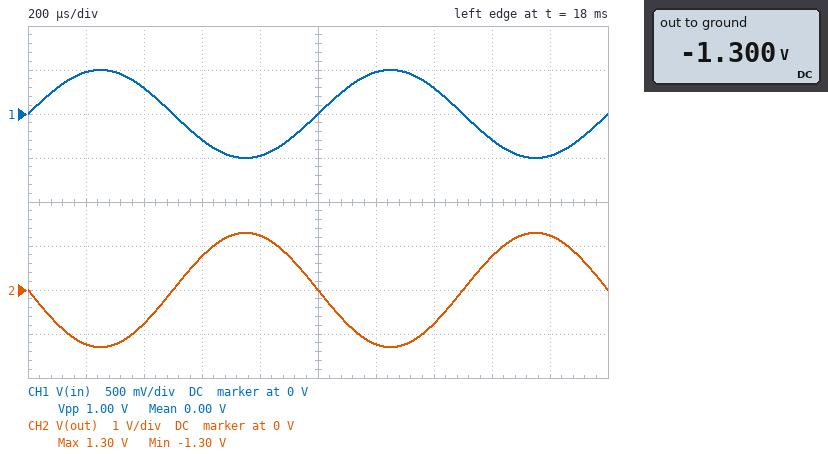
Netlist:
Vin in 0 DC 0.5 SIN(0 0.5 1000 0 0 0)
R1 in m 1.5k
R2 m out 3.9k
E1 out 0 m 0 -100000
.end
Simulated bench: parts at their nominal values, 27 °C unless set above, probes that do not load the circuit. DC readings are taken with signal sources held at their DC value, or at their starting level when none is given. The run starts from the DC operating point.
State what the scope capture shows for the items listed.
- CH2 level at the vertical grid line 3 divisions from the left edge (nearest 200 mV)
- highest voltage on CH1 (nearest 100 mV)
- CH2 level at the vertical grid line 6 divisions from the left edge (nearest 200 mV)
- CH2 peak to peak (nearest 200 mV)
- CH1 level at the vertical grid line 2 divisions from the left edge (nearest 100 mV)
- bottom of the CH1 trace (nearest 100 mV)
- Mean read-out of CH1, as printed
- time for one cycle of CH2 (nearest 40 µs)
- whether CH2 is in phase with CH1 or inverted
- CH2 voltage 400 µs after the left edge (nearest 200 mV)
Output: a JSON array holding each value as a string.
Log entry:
["800 mV", "500 mV", "-1.2 V", "2.6 V", "300 mV", "-500 mV", "0.00 V", "1.00 ms", "inverted", "-800 mV"]
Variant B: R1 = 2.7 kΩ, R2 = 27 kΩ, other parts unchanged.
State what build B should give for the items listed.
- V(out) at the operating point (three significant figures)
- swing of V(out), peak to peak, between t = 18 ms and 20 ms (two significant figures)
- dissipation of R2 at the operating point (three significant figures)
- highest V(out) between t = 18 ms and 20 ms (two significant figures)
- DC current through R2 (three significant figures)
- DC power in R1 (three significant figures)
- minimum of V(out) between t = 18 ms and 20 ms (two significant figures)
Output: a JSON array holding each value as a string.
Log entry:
["-5.00 V", "10 V", "926 µW", "5.0 V", "185 µA", "92.6 µW", "-5.0 V"]
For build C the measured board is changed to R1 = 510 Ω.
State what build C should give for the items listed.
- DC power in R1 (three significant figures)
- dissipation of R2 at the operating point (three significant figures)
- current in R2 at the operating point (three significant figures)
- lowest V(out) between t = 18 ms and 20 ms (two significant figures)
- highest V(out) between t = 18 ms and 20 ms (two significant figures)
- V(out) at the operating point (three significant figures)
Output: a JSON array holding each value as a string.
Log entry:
["490 µW", "3.75 mW", "980 µA", "-3.8 V", "3.8 V", "-3.82 V"]
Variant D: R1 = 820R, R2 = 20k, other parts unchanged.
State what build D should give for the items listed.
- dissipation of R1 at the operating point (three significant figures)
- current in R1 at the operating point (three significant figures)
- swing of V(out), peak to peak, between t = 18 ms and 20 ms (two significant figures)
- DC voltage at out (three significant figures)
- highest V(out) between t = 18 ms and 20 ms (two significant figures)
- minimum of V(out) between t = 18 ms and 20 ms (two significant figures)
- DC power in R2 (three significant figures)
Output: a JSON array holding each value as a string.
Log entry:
["305 µW", "610 µA", "24 V", "-12.2 V", "12 V", "-12 V", "7.43 mW"]
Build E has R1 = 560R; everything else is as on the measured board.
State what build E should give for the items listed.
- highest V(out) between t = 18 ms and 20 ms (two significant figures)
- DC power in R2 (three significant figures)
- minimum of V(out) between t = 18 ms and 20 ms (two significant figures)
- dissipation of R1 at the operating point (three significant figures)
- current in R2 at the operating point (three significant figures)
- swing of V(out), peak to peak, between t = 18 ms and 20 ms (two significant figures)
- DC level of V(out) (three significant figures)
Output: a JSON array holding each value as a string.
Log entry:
["3.5 V", "3.11 mW", "-3.5 V", "446 µW", "893 µA", "7.0 V", "-3.48 V"]
